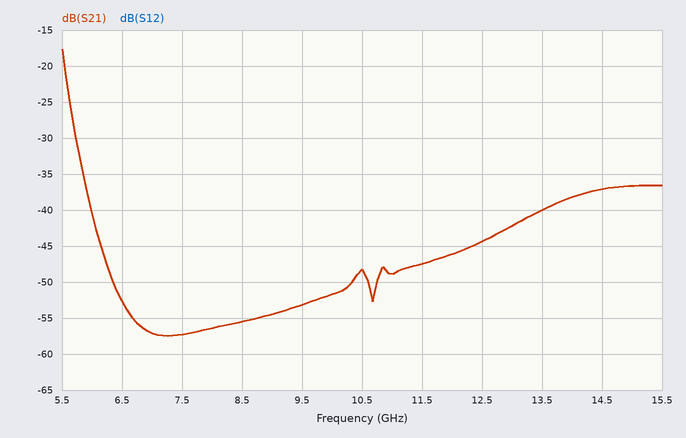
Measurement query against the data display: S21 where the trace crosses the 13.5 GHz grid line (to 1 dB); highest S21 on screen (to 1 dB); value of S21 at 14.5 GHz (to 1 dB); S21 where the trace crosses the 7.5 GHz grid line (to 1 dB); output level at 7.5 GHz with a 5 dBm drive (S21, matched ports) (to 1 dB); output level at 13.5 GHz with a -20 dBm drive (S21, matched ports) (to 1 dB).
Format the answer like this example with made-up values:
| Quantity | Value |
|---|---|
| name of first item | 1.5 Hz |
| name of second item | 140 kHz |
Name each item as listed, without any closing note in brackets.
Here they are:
| Quantity | Value |
|---|---|
| S21 where the trace crosses the 13.5 GHz grid line | -40 dB |
| highest S21 on screen | -18 dB |
| value of S21 at 14.5 GHz | -37 dB |
| S21 where the trace crosses the 7.5 GHz grid line | -57 dB |
| output level at 7.5 GHz with a 5 dBm drive (S21, matched ports) | -52 dBm |
| output level at 13.5 GHz with a -20 dBm drive (S21, matched ports) | -60 dBm |
